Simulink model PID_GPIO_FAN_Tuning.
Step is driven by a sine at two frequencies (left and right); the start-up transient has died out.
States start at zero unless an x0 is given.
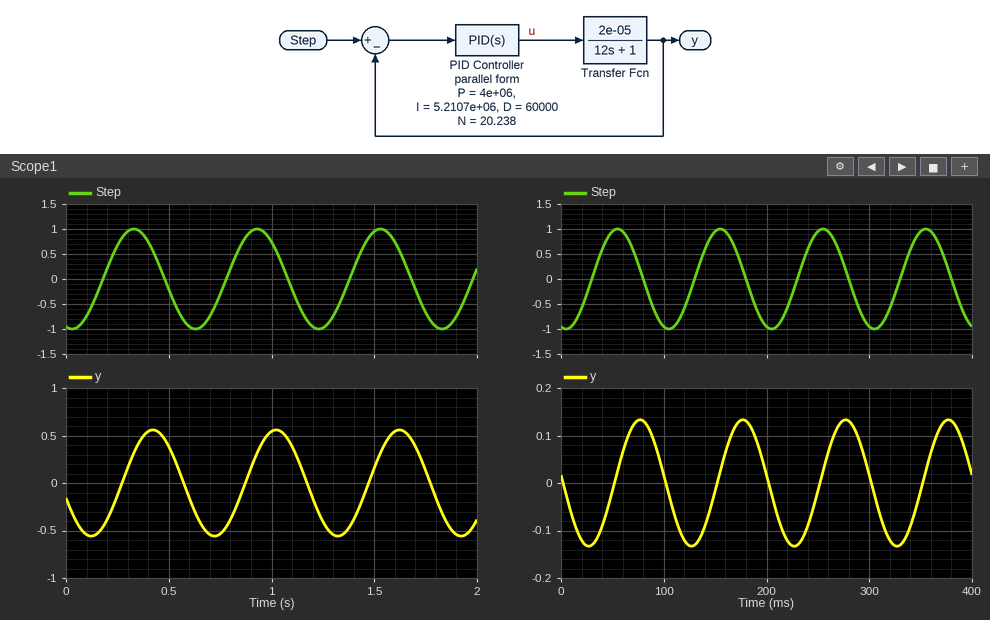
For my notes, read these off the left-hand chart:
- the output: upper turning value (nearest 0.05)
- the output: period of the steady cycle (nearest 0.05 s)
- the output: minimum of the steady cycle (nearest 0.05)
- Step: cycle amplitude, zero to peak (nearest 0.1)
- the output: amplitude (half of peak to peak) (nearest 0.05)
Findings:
0.55
0.60 s
-0.55
1.0
0.55
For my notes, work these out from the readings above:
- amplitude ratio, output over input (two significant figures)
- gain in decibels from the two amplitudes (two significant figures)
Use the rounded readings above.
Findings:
0.55
-5.2 dB
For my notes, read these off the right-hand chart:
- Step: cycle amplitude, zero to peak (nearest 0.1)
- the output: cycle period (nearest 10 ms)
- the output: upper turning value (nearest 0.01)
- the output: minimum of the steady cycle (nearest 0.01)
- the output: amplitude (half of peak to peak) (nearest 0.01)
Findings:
1.0
100 ms
0.13
-0.13
0.13
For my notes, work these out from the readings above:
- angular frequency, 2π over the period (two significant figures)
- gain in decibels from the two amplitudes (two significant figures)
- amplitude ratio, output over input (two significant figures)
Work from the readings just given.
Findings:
0.063 rad/ms
-18 dB
0.13
